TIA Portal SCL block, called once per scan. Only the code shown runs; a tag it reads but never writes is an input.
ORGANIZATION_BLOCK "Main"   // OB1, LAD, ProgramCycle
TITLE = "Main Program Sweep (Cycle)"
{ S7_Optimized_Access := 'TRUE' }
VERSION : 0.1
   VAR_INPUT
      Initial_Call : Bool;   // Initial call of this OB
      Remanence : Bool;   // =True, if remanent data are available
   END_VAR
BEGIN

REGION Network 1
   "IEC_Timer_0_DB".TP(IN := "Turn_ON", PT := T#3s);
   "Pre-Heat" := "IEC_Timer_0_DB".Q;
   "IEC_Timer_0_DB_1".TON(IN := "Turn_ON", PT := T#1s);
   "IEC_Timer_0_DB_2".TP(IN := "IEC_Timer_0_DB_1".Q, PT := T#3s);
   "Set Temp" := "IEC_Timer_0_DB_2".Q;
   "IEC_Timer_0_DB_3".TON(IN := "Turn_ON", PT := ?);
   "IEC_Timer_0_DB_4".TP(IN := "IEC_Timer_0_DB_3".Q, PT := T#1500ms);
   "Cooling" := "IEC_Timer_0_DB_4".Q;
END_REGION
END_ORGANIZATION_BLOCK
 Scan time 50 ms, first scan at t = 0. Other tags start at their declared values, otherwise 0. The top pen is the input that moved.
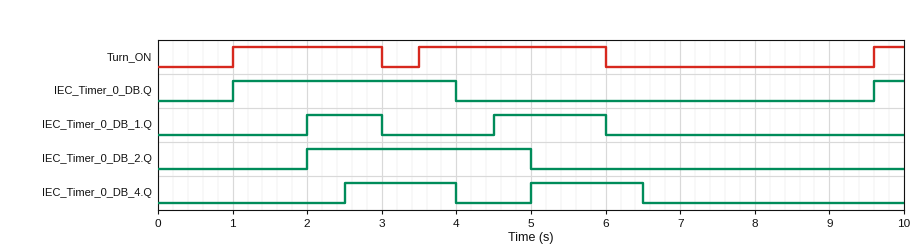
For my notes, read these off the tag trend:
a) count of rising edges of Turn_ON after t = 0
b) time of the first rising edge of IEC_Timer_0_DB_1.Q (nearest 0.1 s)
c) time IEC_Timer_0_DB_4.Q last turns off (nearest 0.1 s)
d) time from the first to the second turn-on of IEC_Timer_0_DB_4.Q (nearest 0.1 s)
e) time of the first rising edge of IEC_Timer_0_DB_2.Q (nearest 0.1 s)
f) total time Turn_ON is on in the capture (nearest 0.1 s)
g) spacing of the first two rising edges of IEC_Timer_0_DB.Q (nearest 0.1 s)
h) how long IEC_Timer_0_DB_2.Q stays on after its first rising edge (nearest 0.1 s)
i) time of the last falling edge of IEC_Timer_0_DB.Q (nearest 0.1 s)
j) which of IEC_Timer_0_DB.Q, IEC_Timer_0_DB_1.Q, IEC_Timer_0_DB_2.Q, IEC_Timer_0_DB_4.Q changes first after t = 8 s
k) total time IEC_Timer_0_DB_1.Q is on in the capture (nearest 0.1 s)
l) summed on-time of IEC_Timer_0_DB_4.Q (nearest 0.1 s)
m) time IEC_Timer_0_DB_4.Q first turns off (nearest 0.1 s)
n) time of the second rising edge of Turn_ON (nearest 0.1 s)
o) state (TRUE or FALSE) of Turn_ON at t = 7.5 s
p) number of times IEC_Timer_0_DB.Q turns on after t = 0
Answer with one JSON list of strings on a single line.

["3", "2.0 s", "6.5 s", "2.5 s", "2.0 s", "4.9 s", "8.6 s", "3.0 s", "4.0 s", "IEC_Timer_0_DB.Q", "2.5 s", "3.0 s", "4.0 s", "3.5 s", "FALSE", "2"]
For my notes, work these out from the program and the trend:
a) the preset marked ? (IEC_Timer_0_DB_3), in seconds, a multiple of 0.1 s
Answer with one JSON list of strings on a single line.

["1.5 s"]
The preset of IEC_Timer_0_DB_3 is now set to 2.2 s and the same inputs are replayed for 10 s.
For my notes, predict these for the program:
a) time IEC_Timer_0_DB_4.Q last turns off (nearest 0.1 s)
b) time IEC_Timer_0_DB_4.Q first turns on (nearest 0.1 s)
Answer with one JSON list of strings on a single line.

["7.2 s", "5.7 s"]
